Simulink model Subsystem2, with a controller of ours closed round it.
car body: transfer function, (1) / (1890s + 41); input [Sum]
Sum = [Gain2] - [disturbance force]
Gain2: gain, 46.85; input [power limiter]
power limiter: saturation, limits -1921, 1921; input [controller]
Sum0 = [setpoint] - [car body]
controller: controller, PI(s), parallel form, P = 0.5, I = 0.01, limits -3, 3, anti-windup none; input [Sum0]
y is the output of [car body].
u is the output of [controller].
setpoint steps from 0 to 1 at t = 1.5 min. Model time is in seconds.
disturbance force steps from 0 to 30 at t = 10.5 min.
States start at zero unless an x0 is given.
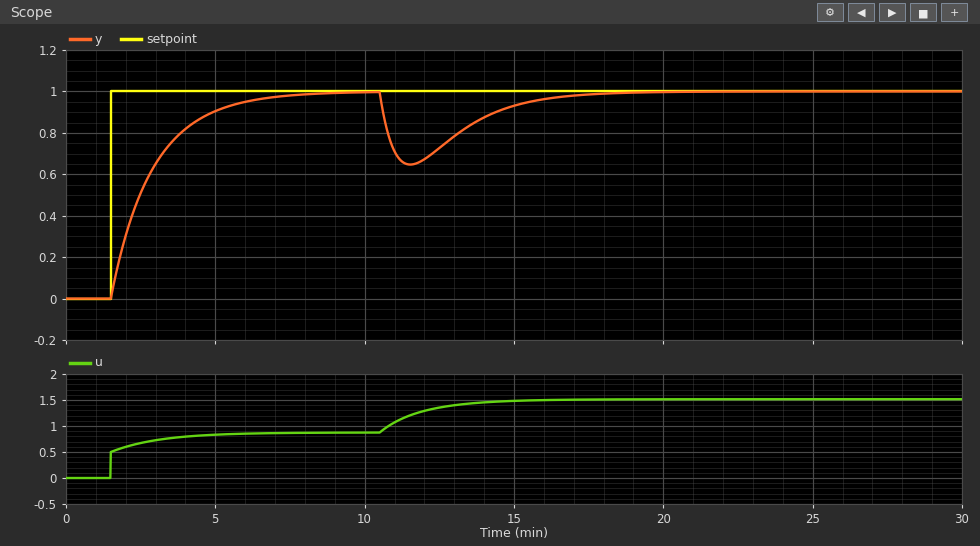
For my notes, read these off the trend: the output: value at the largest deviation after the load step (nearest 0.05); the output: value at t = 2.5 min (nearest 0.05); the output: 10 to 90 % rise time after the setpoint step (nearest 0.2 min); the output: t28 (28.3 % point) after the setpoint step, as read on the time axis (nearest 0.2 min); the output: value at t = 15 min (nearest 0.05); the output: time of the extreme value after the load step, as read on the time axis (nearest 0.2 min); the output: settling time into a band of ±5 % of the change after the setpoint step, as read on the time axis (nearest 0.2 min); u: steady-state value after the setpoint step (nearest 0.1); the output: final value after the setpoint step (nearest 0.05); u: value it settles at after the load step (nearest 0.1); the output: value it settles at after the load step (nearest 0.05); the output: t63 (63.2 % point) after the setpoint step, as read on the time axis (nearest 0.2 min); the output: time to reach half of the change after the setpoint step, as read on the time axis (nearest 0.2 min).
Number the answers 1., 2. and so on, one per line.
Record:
1. 0.65
2. 0.50
3. 3.2 min
4. 2.0 min
5. 0.95
6. 11.6 min
7. 6.0 min
8. 0.9
9. 1.00
10. 1.5
11. 1.00
12. 3.0 min
13. 2.4 min
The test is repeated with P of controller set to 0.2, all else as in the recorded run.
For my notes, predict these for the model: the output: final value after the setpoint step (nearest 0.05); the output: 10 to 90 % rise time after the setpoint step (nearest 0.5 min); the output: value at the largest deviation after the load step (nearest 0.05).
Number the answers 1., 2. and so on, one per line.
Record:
1. 1.00
2. 2.5 min
3. 0.60
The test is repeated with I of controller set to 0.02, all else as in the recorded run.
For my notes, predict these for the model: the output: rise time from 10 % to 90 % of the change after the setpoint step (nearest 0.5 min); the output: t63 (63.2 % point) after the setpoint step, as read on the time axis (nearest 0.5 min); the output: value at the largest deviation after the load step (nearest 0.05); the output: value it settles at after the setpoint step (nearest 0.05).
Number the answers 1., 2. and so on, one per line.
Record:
1. 1.5 min
2. 2.5 min
3. 0.70
4. 1.00
